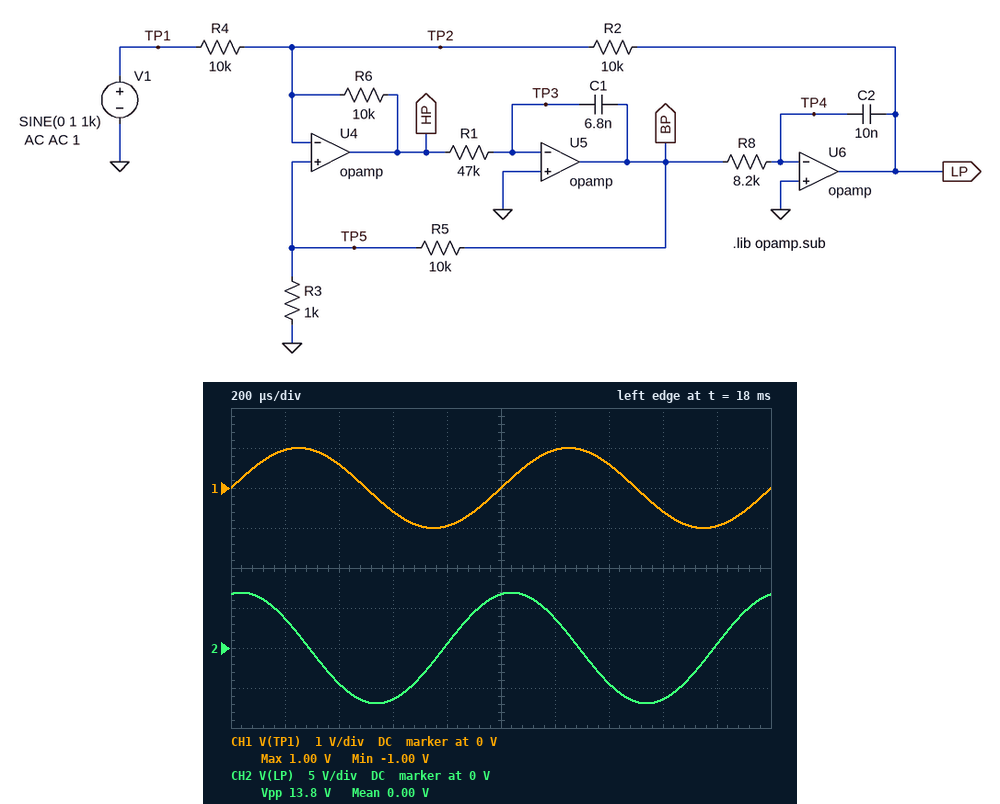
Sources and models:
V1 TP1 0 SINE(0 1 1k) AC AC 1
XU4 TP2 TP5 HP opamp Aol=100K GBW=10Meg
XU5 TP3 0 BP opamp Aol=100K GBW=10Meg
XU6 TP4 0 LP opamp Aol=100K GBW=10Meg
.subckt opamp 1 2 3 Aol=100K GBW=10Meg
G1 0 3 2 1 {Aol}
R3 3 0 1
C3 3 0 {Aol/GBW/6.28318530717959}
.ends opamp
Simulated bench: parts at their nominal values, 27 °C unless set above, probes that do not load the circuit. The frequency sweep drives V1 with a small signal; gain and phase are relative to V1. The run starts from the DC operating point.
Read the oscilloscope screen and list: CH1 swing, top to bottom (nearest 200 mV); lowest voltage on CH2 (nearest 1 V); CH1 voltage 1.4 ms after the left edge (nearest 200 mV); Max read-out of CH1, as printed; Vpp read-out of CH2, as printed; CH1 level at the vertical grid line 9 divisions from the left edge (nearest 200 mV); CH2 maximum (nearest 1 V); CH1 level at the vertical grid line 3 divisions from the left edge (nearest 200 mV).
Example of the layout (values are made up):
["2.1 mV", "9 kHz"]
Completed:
["2.0 V", "-7 V", "600 mV", "1.00 V", "13.8 V", "-1.0 V", "7 V", "-600 mV"]
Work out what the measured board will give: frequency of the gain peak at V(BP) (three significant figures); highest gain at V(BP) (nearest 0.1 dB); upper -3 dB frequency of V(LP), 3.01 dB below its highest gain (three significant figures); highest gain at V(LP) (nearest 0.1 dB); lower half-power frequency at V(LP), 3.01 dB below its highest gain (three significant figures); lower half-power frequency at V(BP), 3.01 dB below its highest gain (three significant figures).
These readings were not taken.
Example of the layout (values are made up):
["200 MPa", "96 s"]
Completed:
["983 Hz", "11.3 dB", "1.04 kHz", "17.2 dB", "908 Hz", "918 Hz"]
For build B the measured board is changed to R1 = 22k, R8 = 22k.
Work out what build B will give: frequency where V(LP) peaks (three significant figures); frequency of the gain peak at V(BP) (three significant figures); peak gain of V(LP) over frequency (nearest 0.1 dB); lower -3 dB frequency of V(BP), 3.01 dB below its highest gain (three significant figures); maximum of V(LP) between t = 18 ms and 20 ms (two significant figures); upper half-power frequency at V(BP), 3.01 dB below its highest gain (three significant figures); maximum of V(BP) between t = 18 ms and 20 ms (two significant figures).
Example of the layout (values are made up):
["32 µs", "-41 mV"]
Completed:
["853 Hz", "877 Hz", "9.7 dB", "744 Hz", "2.1 V", "1.03 kHz", "2.9 V"]
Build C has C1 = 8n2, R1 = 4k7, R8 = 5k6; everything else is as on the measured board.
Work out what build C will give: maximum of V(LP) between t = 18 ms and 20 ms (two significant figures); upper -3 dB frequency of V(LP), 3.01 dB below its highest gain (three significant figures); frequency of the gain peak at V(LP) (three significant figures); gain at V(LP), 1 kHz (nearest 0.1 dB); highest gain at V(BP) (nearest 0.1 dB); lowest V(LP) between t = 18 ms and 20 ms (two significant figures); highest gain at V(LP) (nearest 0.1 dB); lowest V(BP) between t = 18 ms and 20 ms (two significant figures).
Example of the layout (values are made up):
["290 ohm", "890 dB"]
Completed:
["1.1 V", "3.86 kHz", "3.33 kHz", "0.7 dB", "11.3 dB", "-1.1 V", "9.8 dB", "-380 mV"]
